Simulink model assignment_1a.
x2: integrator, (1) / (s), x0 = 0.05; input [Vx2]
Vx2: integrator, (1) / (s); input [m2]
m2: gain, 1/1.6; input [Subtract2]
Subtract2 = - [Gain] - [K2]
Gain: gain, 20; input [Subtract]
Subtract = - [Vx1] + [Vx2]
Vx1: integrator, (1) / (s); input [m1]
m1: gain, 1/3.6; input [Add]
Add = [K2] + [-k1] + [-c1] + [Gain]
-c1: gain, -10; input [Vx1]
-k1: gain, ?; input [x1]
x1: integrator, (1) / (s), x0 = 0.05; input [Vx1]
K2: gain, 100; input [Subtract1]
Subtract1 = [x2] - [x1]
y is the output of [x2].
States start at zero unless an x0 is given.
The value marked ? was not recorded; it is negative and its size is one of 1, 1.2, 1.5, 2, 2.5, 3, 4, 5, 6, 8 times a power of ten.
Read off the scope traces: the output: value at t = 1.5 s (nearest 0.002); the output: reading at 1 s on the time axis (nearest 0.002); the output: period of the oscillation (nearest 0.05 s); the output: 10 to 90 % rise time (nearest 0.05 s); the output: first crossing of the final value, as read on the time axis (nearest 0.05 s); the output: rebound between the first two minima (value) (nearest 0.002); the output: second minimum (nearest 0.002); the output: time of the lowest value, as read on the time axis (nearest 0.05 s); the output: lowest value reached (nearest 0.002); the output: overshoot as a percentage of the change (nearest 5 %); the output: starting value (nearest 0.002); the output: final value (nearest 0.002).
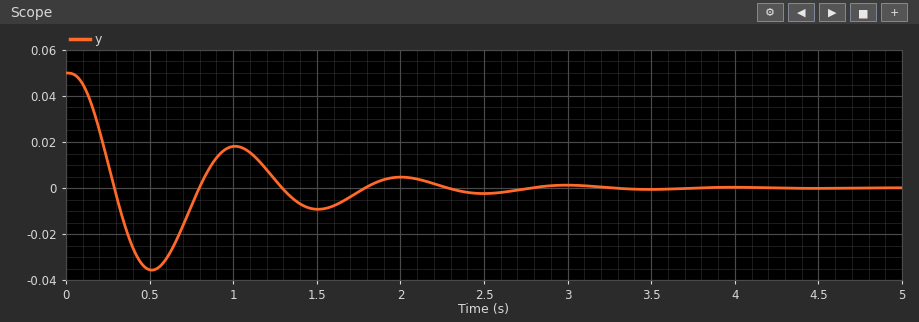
-0.010
0.018
1.00 s
0.15 s
0.30 s
0.018
-0.010
0.50 s
-0.036
70 %
0.050
0.000
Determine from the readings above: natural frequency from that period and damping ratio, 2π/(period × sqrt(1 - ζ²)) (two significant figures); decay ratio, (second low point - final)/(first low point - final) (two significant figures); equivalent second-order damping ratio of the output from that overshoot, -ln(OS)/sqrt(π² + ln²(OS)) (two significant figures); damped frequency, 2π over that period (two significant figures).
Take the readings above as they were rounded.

6.3 rad/s
0.28
0.11
6.3 rad/s
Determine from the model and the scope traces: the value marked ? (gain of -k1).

-250
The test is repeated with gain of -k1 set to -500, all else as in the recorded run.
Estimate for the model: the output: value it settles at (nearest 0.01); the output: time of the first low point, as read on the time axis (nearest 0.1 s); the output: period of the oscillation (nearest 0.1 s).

0.00
0.4 s
0.7 s
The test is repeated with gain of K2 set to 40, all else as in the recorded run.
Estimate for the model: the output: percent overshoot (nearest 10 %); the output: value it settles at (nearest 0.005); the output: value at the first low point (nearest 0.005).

60 %
0.000
-0.030
